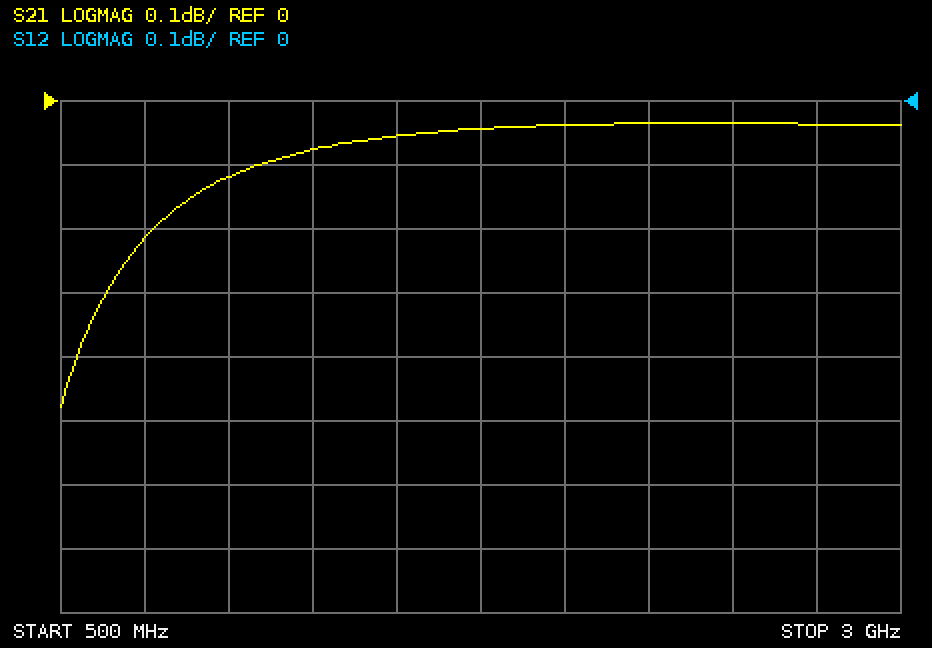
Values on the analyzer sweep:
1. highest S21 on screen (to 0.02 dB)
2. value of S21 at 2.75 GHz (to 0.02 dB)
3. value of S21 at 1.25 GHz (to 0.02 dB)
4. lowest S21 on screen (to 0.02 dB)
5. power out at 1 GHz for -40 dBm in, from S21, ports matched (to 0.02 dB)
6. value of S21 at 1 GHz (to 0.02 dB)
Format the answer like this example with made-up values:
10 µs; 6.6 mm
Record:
-0.04 dB; -0.04 dB; -0.08 dB; -0.48 dB; -40.12 dBm; -0.12 dB
